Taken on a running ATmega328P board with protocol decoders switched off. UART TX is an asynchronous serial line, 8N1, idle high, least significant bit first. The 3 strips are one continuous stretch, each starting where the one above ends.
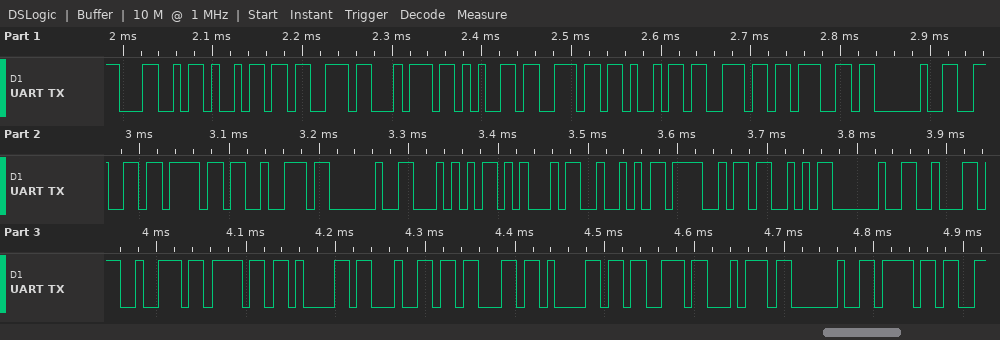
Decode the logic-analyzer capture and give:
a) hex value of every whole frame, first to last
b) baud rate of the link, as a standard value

4C 69 73 74 65 6E 69 6E 67 20 66 6F 72 20 54 45 52 4F 53 20 62 72 6F 61 64 63 61 73 74 20 6F
115200 baud
